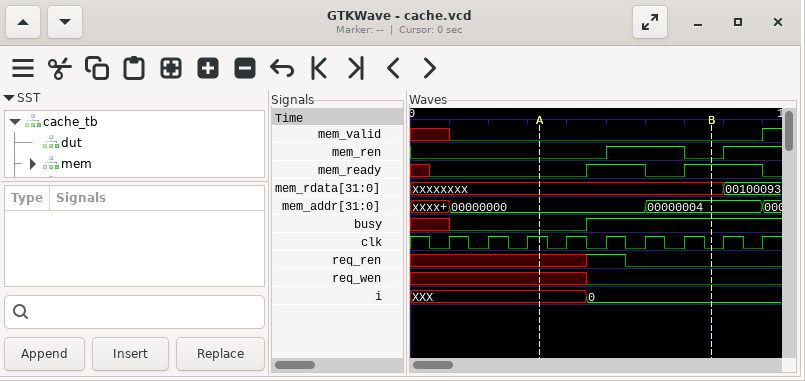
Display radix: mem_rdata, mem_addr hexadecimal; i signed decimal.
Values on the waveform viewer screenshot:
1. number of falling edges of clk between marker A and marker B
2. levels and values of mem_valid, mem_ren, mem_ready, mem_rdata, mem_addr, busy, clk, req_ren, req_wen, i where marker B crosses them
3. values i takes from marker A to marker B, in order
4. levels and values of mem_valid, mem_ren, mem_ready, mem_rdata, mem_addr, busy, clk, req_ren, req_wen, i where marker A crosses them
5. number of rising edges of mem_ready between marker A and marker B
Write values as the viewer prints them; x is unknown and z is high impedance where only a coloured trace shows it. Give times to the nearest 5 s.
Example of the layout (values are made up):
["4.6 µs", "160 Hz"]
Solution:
["5", "mem_valid=0, mem_ren=0, mem_ready=1, mem_rdata=xxxxxxxx, mem_addr=00000004, busy=1, clk=0, req_ren=0, req_wen=0, i=0", "XXX, 0", "mem_valid=0, mem_ren=0, mem_ready=0, mem_rdata=xxxxxxxx, mem_addr=00000000, busy=0, clk=1, req_ren=x, req_wen=x, i=XXX", "2"]
